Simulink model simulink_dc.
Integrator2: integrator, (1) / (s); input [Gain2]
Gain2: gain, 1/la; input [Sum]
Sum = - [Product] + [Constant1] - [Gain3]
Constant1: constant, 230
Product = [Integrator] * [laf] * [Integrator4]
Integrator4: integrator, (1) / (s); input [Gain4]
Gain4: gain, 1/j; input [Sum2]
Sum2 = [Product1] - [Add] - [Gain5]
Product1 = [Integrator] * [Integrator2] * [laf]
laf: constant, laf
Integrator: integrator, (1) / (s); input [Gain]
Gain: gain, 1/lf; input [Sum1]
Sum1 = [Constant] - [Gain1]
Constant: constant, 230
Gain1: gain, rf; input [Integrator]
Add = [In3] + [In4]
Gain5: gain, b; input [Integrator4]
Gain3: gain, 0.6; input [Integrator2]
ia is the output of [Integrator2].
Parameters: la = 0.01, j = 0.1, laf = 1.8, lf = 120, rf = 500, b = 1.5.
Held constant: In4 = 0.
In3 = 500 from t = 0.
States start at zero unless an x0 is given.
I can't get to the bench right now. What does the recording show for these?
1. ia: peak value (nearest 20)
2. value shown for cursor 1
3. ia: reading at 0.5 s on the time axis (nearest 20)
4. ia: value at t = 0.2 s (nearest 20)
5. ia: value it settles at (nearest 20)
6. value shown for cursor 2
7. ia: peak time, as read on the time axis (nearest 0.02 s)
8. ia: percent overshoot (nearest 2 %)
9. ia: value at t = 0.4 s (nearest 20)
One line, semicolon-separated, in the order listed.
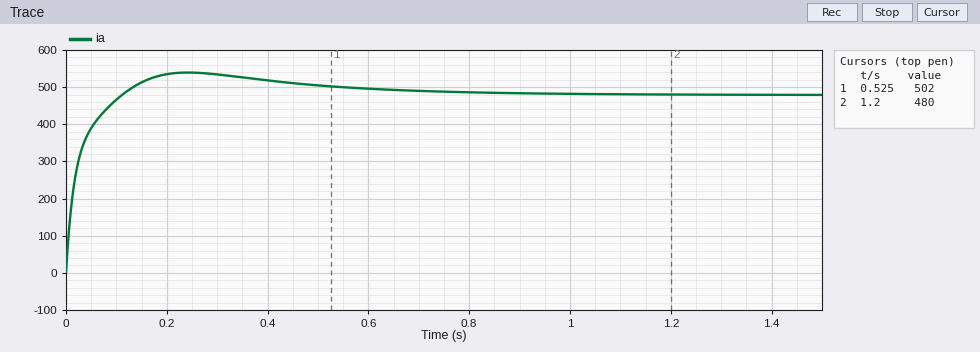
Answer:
540; 502; 500; 540; 480; 480; 0.24 s; 12 %; 520
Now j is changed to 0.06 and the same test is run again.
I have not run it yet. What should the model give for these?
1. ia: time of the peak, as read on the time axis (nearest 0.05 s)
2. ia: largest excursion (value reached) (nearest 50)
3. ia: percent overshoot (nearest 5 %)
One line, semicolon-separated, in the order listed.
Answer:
0.20 s; 550; 10 %
